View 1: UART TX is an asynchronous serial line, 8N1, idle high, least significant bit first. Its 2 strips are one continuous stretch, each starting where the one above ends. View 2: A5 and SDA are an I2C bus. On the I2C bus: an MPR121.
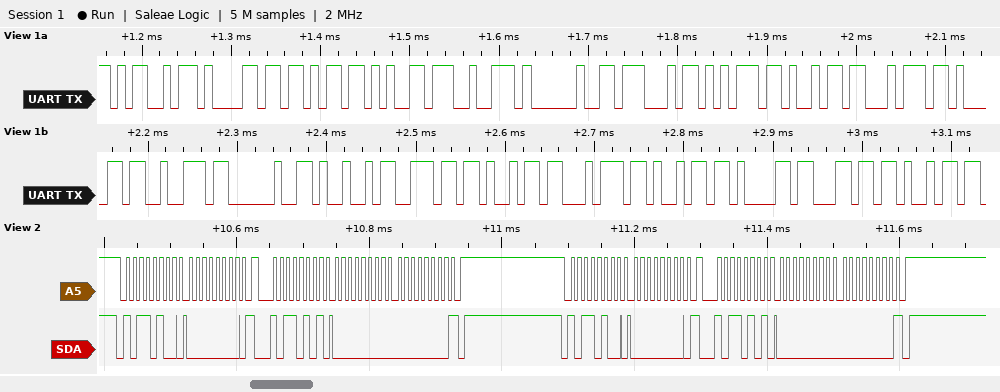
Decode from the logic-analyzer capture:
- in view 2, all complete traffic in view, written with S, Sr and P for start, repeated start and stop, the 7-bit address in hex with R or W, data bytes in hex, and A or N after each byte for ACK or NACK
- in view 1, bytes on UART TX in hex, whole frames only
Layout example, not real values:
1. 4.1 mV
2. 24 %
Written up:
1. S 5AW A 00 A Sr 5AR A 00 A 00 N P S 5AW A 00 A Sr 5AR A 00 A 00 N P
2. 4D 61 6B 65 72 20 47 75 69 74 61 72 20 49 6E 69 74 69 61 6C 69
